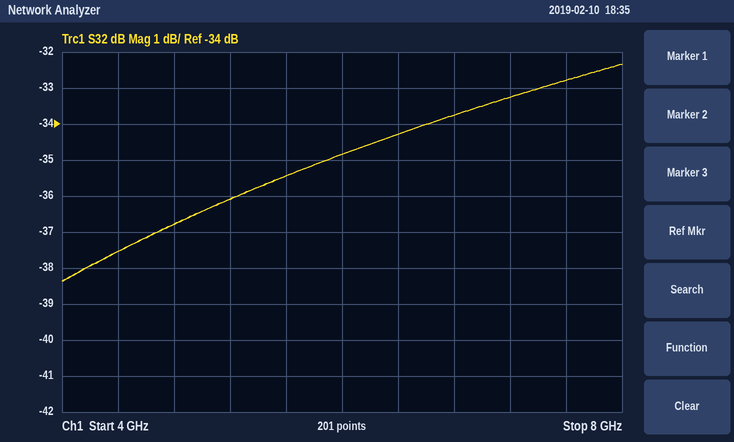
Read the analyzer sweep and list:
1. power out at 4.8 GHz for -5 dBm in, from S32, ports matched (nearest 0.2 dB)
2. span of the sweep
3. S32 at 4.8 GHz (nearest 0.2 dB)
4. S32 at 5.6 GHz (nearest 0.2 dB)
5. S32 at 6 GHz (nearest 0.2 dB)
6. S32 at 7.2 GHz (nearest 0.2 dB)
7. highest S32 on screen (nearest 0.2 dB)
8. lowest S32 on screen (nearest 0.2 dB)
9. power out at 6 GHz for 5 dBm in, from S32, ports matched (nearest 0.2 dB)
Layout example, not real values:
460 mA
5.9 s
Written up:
-41.8 dBm
4 GHz
-36.8 dB
-35.4 dB
-34.8 dB
-33.2 dB
-32.4 dB
-38.4 dB
-29.8 dBm
